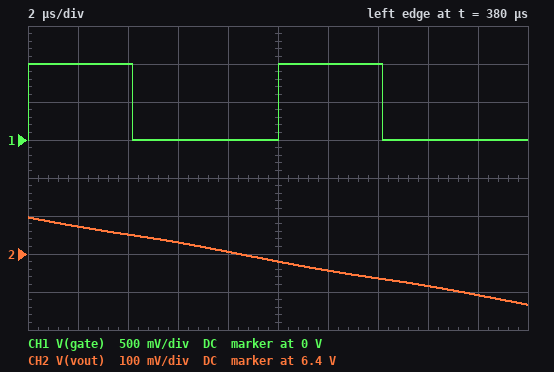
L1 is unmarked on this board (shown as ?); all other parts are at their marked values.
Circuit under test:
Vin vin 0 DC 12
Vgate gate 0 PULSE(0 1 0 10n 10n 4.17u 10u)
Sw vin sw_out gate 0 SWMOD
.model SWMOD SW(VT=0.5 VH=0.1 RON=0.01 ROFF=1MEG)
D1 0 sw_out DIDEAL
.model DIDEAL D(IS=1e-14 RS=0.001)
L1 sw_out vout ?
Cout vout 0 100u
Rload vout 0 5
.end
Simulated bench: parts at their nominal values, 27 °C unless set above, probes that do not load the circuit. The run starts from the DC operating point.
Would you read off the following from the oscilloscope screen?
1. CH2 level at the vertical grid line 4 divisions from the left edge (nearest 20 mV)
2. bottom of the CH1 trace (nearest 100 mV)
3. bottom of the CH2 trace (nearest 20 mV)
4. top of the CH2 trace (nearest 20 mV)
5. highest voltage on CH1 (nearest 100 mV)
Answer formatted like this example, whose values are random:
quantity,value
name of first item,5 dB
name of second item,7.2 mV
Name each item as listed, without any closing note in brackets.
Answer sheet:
quantity,value
CH2 level at the vertical grid line 4 divisions from the left edge,6.40 V
bottom of the CH1 trace,0 V
bottom of the CH2 trace,6.26 V
top of the CH2 trace,6.50 V
highest voltage on CH1,1.0 V
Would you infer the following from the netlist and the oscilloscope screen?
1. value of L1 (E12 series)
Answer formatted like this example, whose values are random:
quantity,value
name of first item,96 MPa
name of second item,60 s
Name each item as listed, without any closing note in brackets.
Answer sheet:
quantity,value
value of L1,68 µH
